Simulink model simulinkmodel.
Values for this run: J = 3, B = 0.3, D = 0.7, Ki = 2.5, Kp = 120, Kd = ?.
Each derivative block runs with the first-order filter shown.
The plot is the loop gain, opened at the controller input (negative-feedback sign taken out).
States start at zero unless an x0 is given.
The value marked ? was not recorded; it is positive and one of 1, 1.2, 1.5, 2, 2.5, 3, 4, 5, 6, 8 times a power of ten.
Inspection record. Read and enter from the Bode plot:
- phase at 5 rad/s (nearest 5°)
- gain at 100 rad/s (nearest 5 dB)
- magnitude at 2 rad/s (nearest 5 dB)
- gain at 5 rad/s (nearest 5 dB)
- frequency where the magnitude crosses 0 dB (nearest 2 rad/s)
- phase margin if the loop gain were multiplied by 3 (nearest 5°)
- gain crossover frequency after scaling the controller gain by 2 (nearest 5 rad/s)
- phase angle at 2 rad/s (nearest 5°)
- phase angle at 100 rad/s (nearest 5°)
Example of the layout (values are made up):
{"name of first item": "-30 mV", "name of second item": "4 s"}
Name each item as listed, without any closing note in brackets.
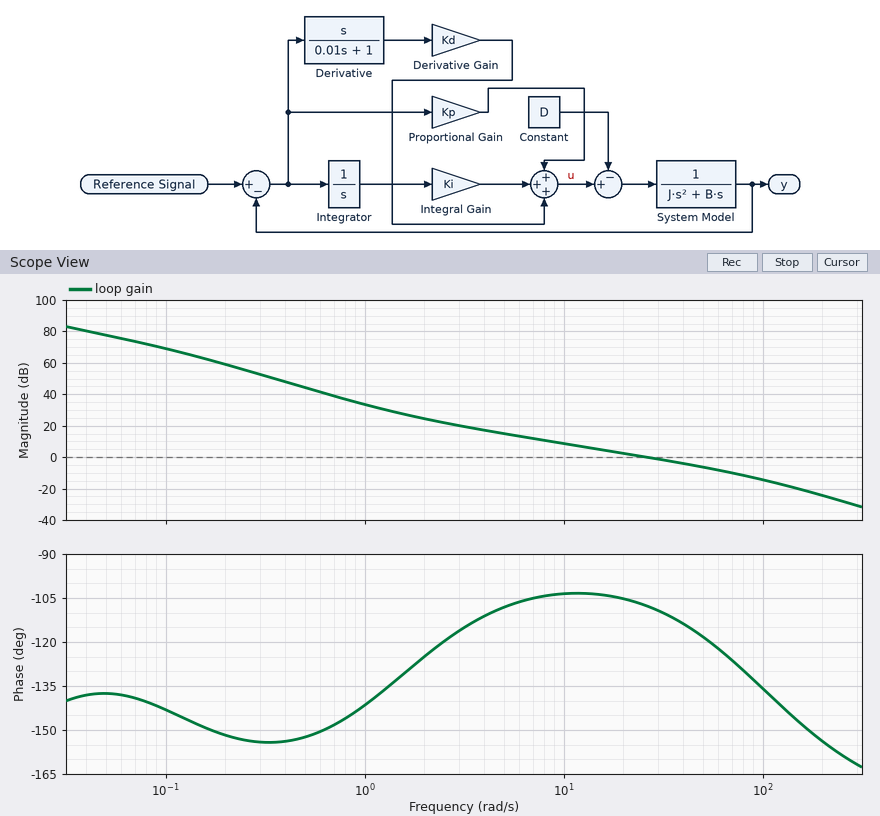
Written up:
{"phase at 5 rad/s": "-110°", "gain at 100 rad/s": "-15 dB", "magnitude at 2 rad/s": "25 dB", "gain at 5 rad/s": "15 dB", "frequency where the magnitude crosses 0 dB": "26 rad/s", "phase margin if the loop gain were multiplied by 3": "55°", "gain crossover frequency after scaling the controller gain by 2": "50 rad/s", "phase angle at 2 rad/s": "-125°", "phase angle at 100 rad/s": "-135°"}
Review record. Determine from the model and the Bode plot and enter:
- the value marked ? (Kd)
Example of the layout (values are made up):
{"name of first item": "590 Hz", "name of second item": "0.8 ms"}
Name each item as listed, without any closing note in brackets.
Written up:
{"the value marked ?": "80"}
